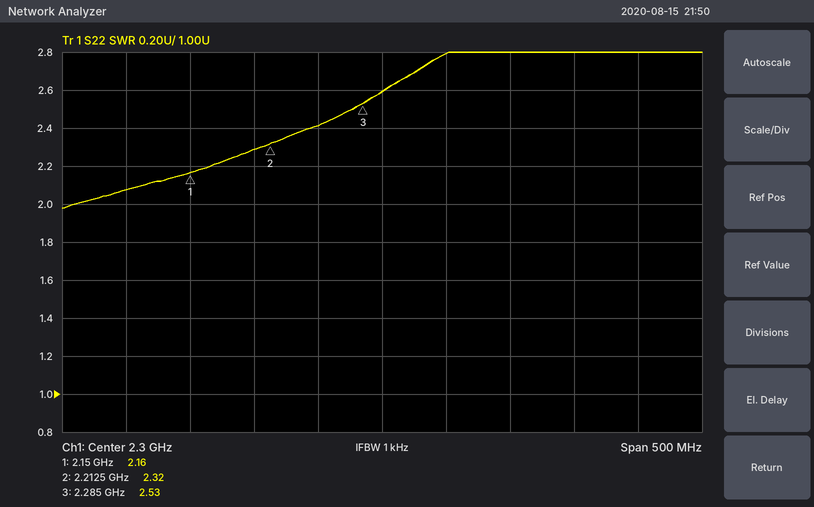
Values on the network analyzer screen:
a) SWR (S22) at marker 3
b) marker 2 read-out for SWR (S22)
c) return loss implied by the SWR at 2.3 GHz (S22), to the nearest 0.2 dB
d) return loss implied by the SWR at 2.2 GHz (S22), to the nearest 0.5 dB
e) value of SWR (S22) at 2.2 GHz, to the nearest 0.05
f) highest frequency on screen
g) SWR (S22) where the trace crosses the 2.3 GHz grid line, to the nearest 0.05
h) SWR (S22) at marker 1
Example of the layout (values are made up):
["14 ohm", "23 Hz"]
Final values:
["2.53", "2.32", "7.0 dB", "8.0 dB", "2.30", "2.55 GHz", "2.60", "2.16"]
